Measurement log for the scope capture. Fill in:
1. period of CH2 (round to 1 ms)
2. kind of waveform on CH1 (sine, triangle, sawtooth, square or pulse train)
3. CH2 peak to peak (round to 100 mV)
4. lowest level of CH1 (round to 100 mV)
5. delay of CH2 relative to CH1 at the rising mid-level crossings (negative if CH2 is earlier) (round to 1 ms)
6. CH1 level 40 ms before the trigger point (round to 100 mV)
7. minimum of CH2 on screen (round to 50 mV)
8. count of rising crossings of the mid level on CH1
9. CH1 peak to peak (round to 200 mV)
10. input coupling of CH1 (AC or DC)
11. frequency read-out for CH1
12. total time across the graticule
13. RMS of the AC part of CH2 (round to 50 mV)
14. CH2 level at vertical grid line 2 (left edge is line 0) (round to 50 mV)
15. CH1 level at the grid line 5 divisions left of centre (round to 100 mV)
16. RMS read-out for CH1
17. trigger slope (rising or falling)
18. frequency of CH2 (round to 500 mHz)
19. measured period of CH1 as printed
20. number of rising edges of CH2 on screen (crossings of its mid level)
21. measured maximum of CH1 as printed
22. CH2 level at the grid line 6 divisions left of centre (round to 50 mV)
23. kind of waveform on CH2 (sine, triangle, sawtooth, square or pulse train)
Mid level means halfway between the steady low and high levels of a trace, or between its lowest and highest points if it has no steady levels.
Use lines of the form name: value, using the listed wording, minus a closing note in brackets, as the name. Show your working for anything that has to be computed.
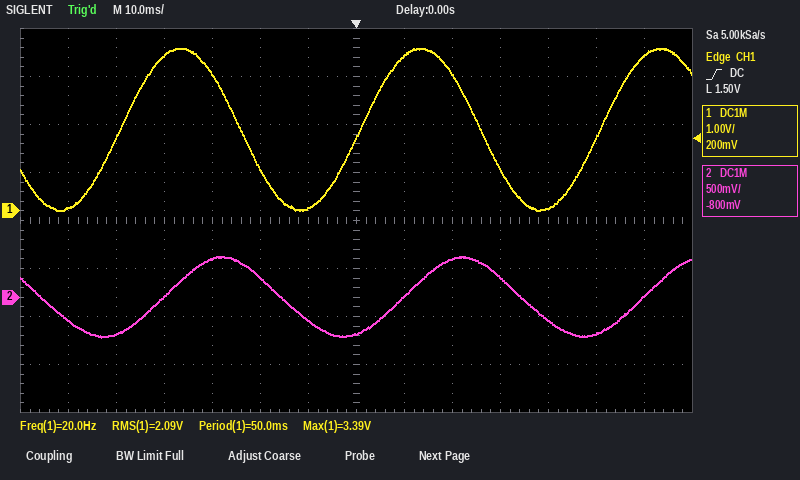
period of CH2: 50 ms
kind of waveform on CH1: sine
CH2 peak to peak: 800 mV
lowest level of CH1: 0.0 V
delay of CH2 relative to CH1 at the rising mid-level crossings (negative if CH2 is earlier): +9 ms
CH1 level 40 ms before the trigger point: 3.2 V
minimum of CH2 on screen: -400 mV
count of rising crossings of the mid level on CH1: 3
CH1 peak to peak: 3.4 V
input coupling of CH1: DC
frequency read-out for CH1: 20.0 Hz
total time across the graticule: 140 ms
RMS of the AC part of CH2: 800 mV / (2√2) ≈ 283 mV, so 300 mV to the nearest 50 mV
CH2 level at vertical grid line 2 (left edge is line 0): -400 mV
CH1 level at the grid line 5 divisions left of centre: 1.5 V
RMS read-out for CH1: 2.09 V
trigger slope: rising
frequency of CH2: 1 / 50 ms ≈ 20.0 Hz
measured period of CH1 as printed: 50.0 ms
number of rising edges of CH2 on screen: 3
measured maximum of CH1 as printed: 3.39 V
CH2 level at the grid line 6 divisions left of centre: -250 mV
kind of waveform on CH2: sine
